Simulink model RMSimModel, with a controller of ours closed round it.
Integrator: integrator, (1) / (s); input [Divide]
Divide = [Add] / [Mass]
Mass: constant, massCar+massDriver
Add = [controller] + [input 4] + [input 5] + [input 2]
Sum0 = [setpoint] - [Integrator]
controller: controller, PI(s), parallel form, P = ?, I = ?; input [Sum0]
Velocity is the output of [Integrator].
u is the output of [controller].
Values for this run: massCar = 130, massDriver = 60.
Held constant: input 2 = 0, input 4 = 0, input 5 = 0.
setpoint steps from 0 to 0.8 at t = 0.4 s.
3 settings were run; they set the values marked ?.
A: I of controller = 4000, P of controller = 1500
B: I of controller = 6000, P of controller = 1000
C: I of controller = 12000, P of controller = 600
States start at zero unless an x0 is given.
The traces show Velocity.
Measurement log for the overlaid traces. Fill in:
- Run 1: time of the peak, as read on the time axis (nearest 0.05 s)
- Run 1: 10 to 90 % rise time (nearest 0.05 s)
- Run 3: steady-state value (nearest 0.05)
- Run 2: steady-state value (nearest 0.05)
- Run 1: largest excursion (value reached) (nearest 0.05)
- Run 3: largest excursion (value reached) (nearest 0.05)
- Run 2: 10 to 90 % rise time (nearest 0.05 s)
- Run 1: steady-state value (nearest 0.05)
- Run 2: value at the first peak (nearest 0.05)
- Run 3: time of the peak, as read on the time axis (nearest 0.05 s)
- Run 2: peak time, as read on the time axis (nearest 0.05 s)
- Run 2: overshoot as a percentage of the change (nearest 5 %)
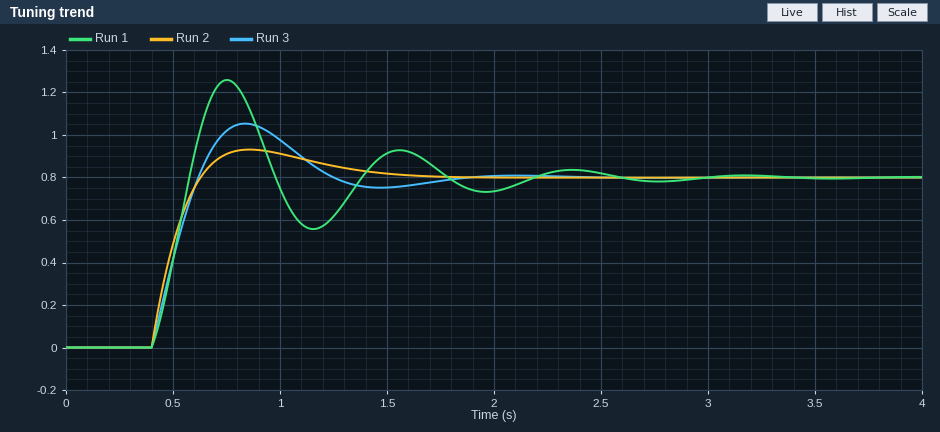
0.75 s
0.15 s
0.80
0.80
1.25
1.05
0.15 s
0.80
0.95
0.85 s
0.85 s
15 %
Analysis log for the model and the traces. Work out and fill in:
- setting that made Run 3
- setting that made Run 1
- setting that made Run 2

B
C
A
